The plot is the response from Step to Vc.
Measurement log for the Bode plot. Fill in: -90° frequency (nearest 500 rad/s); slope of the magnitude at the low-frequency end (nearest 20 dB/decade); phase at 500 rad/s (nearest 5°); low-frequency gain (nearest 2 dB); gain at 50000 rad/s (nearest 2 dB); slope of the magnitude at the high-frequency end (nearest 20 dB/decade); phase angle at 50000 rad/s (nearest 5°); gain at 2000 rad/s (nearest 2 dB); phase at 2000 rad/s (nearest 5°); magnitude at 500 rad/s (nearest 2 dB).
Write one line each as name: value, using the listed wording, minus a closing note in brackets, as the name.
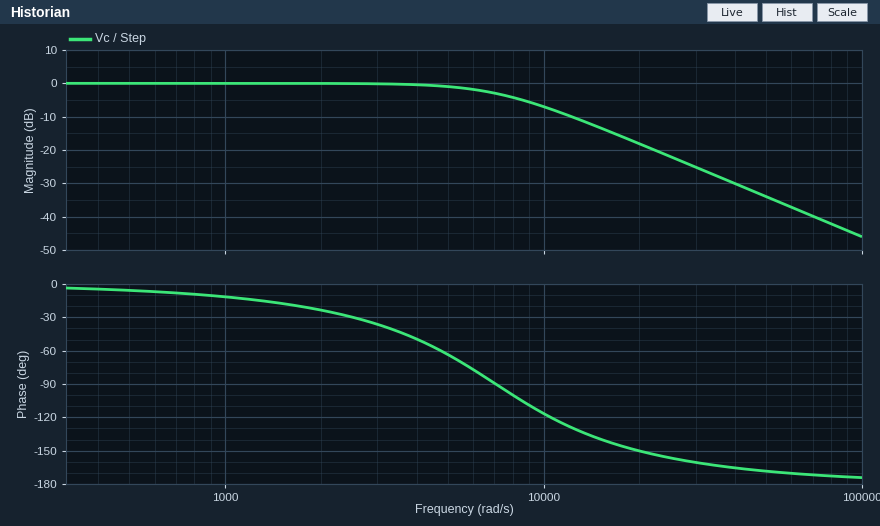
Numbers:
-90° frequency: 7000 rad/s
slope of the magnitude at the low-frequency end: 0 dB/decade
phase at 500 rad/s: -5°
low-frequency gain: 0 dB
gain at 50000 rad/s: -34 dB
slope of the magnitude at the high-frequency end: -40 dB/decade
phase angle at 50000 rad/s: -170°
gain at 2000 rad/s: 0 dB
phase at 2000 rad/s: -25°
magnitude at 500 rad/s: 0 dB
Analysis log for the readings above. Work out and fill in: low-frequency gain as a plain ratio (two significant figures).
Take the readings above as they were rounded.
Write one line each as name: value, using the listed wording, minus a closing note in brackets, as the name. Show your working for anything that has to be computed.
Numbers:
low-frequency gain as a plain ratio: 10^(0 / 20) = 1.0
